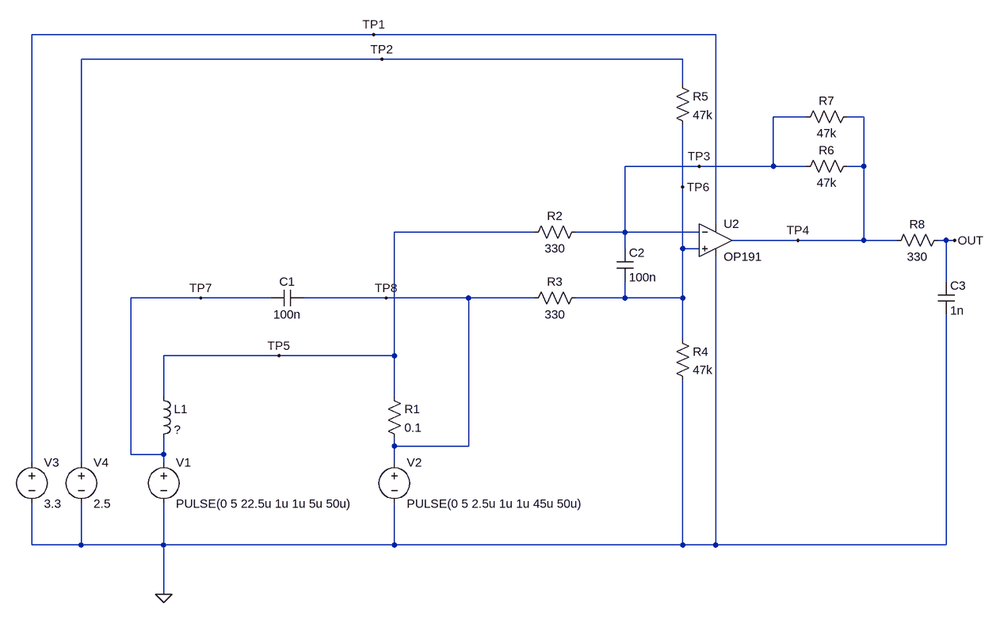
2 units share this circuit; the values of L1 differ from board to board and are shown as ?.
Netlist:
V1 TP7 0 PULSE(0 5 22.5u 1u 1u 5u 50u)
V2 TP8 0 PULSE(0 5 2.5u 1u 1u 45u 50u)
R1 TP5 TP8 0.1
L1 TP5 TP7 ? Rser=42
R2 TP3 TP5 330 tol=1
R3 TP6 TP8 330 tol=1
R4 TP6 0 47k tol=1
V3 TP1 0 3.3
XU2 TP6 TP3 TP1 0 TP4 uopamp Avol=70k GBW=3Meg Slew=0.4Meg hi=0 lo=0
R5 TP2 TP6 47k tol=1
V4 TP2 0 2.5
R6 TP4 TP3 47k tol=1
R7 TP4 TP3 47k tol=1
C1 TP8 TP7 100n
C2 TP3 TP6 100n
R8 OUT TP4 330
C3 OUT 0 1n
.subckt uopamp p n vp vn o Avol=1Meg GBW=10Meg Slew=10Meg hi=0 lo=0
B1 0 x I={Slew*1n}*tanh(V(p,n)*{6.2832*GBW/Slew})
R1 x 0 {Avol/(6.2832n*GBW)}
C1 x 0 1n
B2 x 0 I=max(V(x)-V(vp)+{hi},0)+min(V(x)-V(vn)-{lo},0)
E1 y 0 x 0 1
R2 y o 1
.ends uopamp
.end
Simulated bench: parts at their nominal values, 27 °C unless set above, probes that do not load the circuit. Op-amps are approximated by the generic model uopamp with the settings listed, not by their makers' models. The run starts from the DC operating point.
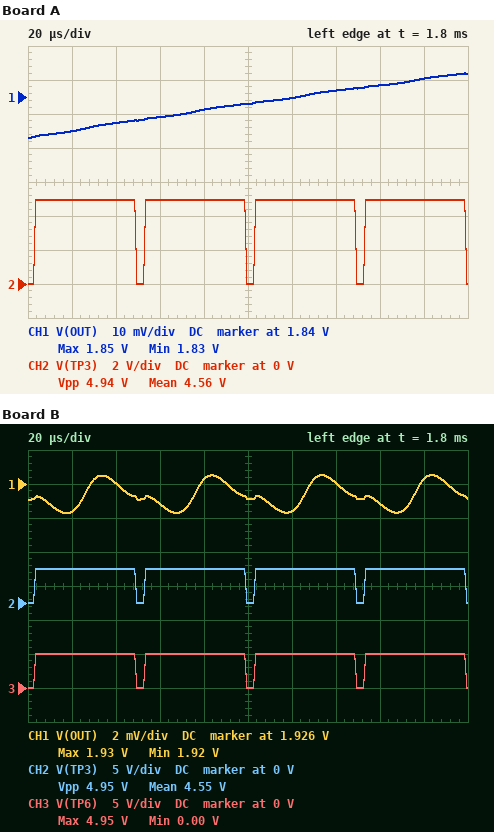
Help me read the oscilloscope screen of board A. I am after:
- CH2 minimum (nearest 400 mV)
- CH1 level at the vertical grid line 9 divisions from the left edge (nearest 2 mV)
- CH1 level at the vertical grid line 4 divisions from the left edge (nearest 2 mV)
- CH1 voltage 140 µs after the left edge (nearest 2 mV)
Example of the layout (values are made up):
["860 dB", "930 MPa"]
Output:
["0 V", "1.846 V", "1.836 V", "1.842 V"]
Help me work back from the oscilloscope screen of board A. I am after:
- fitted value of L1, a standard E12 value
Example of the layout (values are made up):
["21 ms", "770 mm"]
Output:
["39 mH"]
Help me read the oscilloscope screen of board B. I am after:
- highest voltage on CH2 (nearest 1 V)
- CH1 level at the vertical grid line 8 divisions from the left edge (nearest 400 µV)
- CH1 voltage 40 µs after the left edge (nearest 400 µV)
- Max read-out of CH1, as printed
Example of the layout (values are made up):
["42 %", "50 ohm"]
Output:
["5 V", "1.9248 V", "1.9260 V", "1.93 V"]
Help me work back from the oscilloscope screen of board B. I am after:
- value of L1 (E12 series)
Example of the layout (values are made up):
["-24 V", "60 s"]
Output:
["8.2 mH"]
